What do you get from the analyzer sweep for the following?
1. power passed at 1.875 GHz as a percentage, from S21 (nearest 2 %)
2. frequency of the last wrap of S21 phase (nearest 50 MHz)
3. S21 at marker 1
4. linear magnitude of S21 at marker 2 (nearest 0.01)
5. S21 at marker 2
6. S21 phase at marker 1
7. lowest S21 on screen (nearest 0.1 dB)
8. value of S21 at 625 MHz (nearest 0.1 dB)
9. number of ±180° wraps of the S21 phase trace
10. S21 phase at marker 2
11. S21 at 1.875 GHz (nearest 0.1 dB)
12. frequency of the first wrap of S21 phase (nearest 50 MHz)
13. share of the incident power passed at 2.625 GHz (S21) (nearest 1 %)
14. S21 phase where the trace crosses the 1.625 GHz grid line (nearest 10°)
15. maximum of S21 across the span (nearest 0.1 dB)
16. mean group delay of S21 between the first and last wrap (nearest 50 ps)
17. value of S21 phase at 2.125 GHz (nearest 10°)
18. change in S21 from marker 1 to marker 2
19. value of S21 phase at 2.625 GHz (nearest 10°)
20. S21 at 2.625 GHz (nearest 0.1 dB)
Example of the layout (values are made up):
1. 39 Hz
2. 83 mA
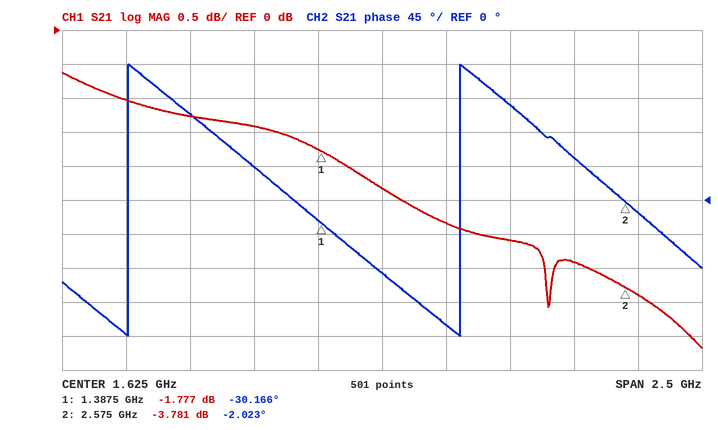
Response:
1. 52 %
2. 1.95 GHz
3. -1.777 dB
4. 0.65
5. -3.781 dB
6. -30.166°
7. -4.7 dB
8. -1.0 dB
9. 2
10. -2.023°
11. -2.8 dB
12. 650 MHz
13. 41 %
14. -100°
15. -0.6 dB
16. 750 ps
17. 130°
18. -2.004 dB
19. -20°
20. -3.9 dB
